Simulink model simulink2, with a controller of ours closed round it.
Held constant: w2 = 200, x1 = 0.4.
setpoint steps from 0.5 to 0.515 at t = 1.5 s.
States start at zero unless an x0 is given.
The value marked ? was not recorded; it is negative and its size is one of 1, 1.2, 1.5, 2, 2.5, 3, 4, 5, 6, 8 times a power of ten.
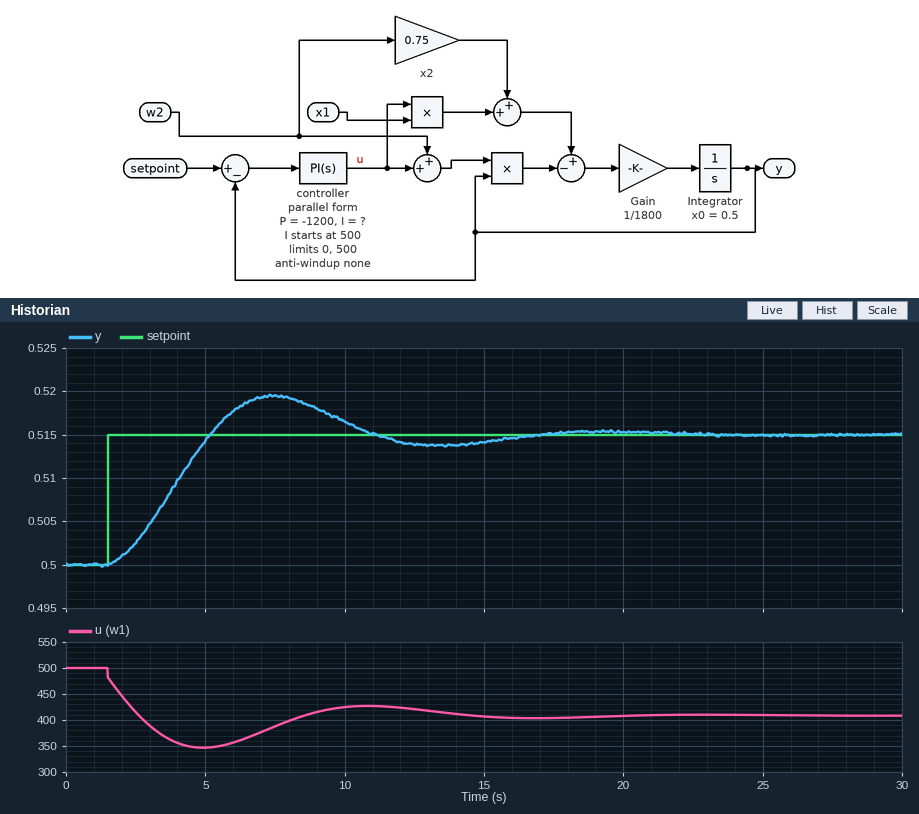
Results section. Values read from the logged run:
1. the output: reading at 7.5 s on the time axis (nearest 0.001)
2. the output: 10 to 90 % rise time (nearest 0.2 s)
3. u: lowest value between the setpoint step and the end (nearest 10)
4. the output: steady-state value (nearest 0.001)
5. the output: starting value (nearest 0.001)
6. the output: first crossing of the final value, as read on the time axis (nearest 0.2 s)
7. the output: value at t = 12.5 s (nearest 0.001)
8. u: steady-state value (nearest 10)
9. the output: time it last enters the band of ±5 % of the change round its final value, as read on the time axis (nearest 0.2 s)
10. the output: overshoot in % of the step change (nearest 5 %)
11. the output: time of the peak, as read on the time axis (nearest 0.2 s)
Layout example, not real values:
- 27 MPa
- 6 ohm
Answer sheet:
- 0.519
- 2.6 s
- 350
- 0.515
- 0.500
- 5.2 s
- 0.514
- 410
- 15.2 s
- 30 %
- 7.4 s
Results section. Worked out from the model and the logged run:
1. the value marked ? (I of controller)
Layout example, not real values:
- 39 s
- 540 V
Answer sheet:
- -5000
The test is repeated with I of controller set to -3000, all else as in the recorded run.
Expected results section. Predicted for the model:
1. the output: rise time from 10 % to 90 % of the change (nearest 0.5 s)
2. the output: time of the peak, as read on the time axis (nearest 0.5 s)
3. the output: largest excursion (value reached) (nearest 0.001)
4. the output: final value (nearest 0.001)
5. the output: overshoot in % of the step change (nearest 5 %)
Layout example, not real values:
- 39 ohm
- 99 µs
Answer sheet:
- 4.0 s
- 9.5 s
- 0.518
- 0.515
- 20 %
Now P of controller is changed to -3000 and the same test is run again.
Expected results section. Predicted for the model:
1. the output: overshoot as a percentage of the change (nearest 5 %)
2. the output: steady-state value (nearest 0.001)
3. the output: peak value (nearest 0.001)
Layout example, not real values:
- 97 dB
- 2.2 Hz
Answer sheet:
- 20 %
- 0.515
- 0.518
